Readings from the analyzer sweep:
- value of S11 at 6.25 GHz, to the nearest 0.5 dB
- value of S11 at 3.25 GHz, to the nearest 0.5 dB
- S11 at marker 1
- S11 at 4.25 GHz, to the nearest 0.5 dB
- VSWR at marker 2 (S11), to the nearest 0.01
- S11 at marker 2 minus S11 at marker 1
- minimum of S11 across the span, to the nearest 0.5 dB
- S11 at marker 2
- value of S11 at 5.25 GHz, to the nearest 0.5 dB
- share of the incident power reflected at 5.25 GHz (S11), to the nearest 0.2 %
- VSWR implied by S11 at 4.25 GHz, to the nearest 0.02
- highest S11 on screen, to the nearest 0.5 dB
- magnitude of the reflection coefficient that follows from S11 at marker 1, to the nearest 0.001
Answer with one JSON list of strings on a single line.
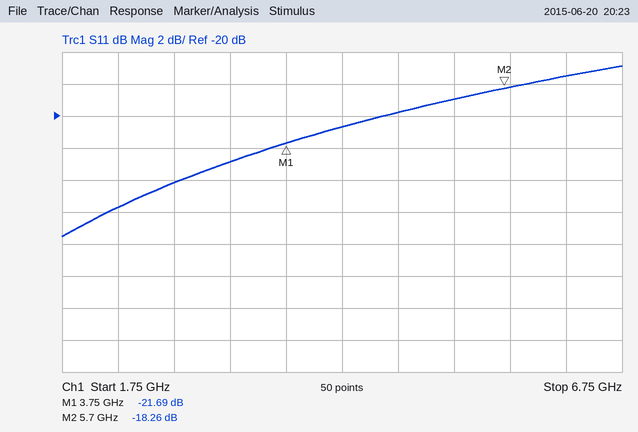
["-17.5 dB", "-23.0 dB", "-21.69 dB", "-20.5 dB", "1.28", "3.43 dB", "-27.5 dB", "-18.26 dB", "-19.0 dB", "1.2 %", "1.20", "-17.0 dB", "0.082"]
